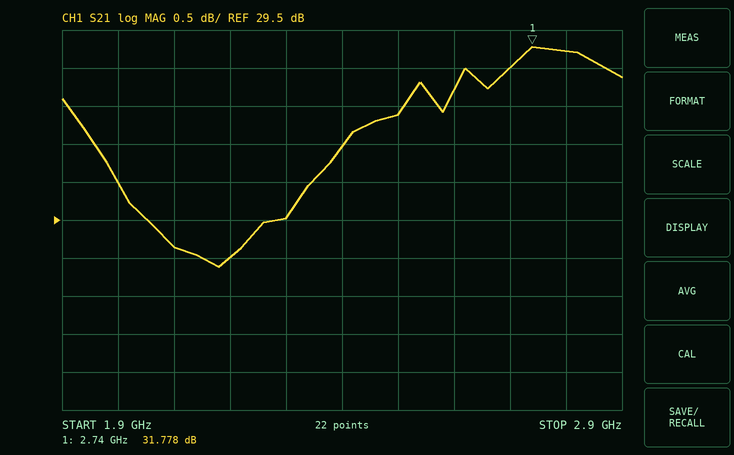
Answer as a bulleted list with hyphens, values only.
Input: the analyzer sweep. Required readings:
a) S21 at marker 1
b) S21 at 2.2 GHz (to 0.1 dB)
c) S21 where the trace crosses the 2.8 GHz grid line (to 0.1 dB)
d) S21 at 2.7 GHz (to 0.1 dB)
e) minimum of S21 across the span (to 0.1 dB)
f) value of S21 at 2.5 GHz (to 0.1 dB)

- 31.778 dB
- 29.0 dB
- 31.7 dB
- 31.5 dB
- 28.9 dB
- 30.9 dB
